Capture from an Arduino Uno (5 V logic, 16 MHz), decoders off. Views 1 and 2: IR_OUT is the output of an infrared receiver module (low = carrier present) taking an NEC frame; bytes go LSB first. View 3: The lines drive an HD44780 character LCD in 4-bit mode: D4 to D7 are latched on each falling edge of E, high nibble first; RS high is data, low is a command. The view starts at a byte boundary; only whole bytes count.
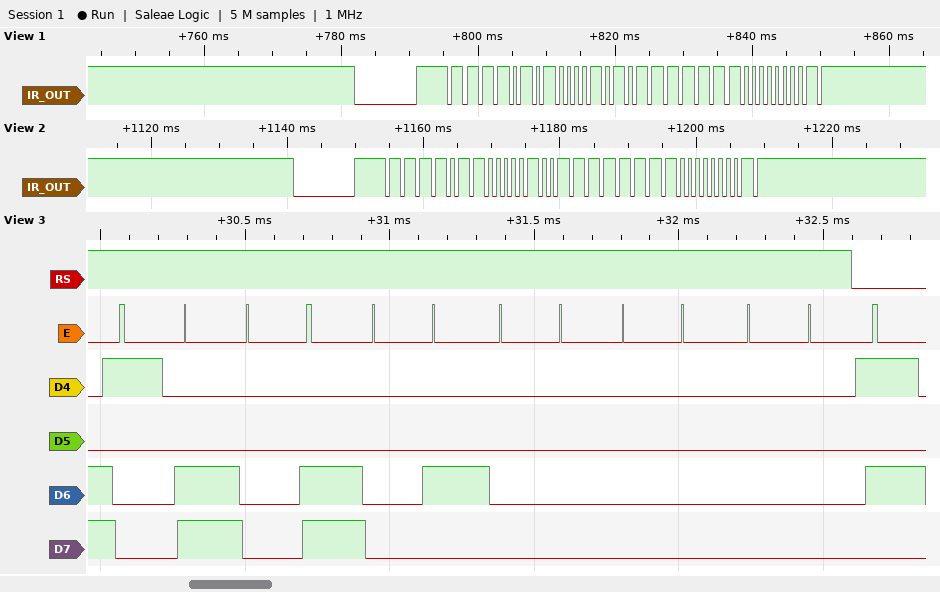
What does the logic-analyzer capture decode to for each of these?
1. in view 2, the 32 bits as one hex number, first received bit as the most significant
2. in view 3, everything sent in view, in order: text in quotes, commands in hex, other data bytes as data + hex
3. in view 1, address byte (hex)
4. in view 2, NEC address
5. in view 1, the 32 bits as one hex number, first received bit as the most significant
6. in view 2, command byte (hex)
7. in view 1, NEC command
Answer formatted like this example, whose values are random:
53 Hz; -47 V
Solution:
0xF609FE01; data 1C 0C 04 00 00 00; 0xAF; 0x6F; 0xF50AFE01; 0x7F; 0x7F
